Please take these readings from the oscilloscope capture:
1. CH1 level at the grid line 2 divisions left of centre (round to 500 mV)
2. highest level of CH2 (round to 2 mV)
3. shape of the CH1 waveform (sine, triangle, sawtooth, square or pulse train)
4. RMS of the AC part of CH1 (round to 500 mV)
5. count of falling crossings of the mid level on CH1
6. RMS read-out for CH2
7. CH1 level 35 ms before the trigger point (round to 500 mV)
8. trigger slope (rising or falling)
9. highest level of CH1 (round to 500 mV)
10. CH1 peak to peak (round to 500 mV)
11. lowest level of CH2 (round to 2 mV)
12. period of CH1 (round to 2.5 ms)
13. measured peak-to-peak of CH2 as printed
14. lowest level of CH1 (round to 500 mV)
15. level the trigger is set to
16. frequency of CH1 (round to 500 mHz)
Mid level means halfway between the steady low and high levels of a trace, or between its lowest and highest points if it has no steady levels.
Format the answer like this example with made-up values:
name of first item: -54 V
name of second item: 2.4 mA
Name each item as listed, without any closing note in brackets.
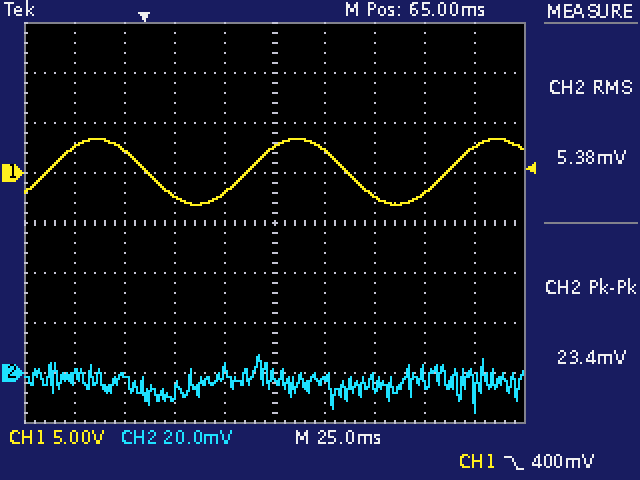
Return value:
CH1 level at the grid line 2 divisions left of centre: -2.5 V
highest level of CH2: 8 mV
shape of the CH1 waveform: sine
RMS of the AC part of CH1: 2.5 V
count of falling crossings of the mid level on CH1: 2
RMS read-out for CH2: 5.38 mV
CH1 level 35 ms before the trigger point: 2.5 V
trigger slope: falling
highest level of CH1: 3.5 V
CH1 peak to peak: 6.5 V
lowest level of CH2: -16 mV
period of CH1: 100.0 ms
measured peak-to-peak of CH2 as printed: 23.4 mV
lowest level of CH1: -3.0 V
level the trigger is set to: 400 mV
frequency of CH1: 10.0 Hz
